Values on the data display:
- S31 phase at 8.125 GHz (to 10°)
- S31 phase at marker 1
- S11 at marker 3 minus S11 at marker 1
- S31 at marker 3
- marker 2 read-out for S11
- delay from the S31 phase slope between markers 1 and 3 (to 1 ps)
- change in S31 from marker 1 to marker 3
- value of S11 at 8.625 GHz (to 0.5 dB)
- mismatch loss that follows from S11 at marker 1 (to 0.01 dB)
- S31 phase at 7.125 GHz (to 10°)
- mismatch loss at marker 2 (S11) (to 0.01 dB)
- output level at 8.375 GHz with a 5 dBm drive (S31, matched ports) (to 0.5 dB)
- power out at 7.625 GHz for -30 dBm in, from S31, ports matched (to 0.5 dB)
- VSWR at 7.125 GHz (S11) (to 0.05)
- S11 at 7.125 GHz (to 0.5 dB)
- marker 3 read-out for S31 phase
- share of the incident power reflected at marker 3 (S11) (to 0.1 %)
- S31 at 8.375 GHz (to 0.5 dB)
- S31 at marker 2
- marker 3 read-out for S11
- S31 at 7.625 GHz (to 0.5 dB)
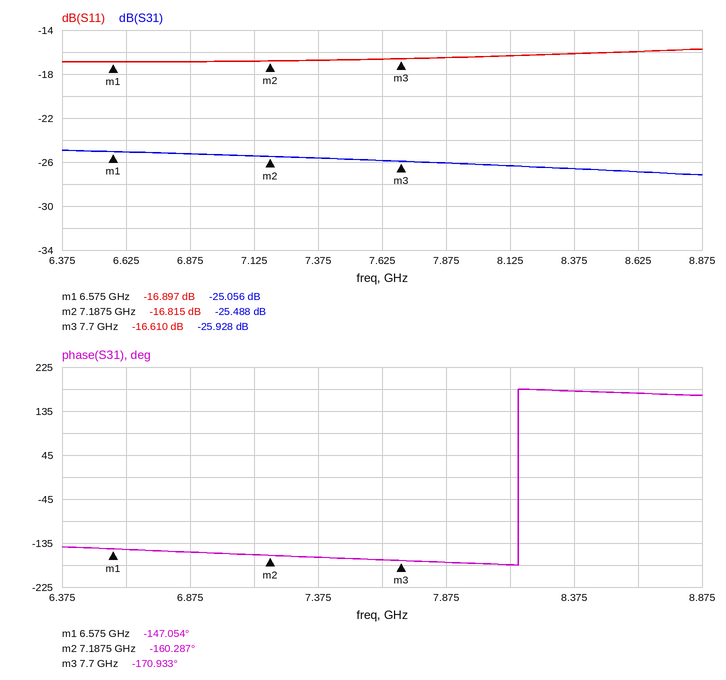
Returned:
-180°
-147.054°
0.287 dB
-25.928 dB
-16.815 dB
59 ps
-0.872 dB
-16.0 dB
0.09 dB
-160°
0.09 dB
-21.5 dBm
-56.0 dBm
1.35
-17.0 dB
-170.933°
2.2 %
-26.5 dB
-25.488 dB
-16.610 dB
-26.0 dB
